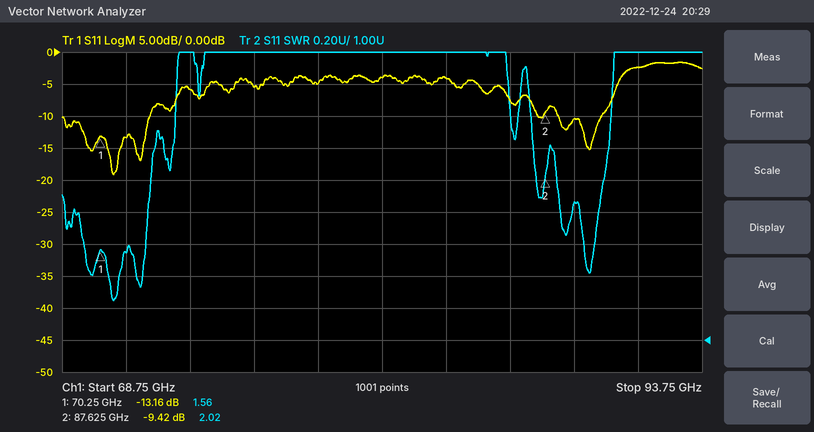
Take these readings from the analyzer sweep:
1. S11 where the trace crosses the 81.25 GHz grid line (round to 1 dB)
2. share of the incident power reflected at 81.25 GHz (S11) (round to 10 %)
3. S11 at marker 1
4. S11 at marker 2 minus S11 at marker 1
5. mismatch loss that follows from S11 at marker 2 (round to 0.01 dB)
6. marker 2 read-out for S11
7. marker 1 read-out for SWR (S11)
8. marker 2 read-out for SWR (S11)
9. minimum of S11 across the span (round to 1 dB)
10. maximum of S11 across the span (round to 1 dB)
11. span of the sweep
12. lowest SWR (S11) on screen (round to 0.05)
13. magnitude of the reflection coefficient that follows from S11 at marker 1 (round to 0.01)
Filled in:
-4 dB
40 %
-13.16 dB
3.74 dB
0.53 dB
-9.42 dB
1.56
2.02
-19 dB
-2 dB
25 GHz
1.25
0.22
